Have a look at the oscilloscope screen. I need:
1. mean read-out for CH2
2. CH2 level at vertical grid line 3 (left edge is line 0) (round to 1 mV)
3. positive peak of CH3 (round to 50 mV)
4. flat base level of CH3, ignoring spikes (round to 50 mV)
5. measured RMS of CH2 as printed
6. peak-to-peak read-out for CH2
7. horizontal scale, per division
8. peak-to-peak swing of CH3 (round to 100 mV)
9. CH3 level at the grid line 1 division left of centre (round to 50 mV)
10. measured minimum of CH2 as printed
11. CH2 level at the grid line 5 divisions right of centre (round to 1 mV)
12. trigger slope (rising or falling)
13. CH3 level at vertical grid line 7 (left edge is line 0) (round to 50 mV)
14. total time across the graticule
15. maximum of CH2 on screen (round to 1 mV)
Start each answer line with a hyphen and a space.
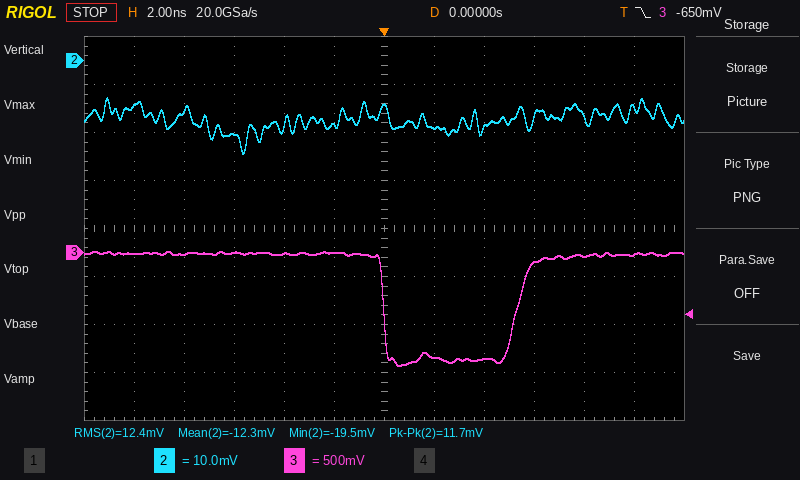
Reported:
- -12.3 mV
- -15 mV
- 0 mV
- -1.10 V
- 12.4 mV
- 11.7 mV
- 2 ns
- 1.20 V
- 0 mV
- -19.5 mV
- -10 mV
- falling
- -1.10 V
- 24 ns
- -8 mV
